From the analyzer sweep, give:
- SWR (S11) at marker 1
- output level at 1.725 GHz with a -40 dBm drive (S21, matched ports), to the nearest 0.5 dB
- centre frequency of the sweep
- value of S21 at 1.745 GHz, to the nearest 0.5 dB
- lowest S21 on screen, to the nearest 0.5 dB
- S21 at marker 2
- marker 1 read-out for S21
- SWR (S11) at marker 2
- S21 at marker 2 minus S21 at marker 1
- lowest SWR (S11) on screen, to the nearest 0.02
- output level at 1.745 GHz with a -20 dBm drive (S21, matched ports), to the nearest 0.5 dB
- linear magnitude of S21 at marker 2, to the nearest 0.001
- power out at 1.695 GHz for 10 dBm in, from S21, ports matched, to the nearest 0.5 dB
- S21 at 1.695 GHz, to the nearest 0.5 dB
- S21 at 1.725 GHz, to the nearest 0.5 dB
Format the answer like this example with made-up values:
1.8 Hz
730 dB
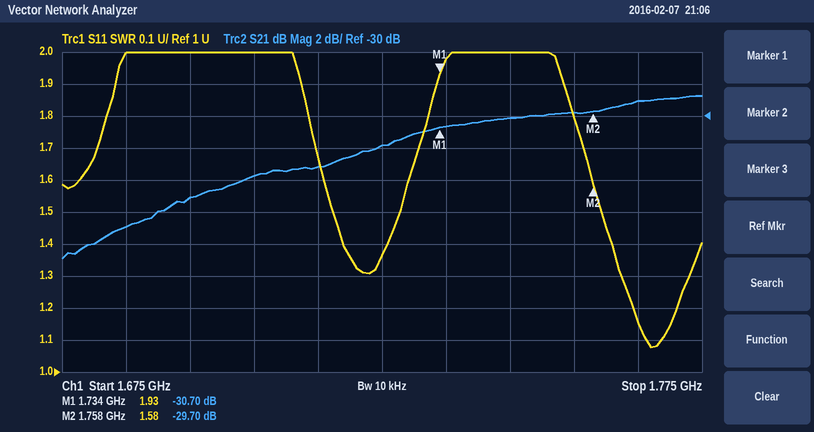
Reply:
1.93
-72.0 dBm
1.725 GHz
-30.0 dB
-39.0 dB
-29.70 dB
-30.70 dB
1.58
1.00 dB
1.08
-50.0 dBm
0.033
-25.0 dBm
-35.0 dB
-32.0 dB
